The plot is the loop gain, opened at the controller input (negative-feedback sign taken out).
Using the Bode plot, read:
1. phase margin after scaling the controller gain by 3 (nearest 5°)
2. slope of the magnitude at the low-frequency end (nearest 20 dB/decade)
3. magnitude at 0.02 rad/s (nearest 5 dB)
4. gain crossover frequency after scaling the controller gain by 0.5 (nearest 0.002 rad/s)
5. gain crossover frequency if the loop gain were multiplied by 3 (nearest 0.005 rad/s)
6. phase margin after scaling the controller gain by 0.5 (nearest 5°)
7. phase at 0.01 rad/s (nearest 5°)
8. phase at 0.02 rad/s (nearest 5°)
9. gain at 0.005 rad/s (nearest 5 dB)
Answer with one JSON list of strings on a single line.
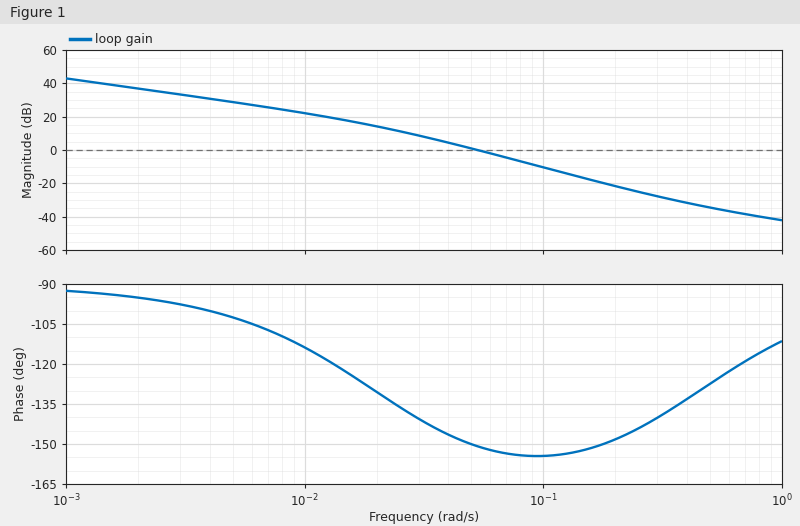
["25°", "-20 dB/decade", "15 dB", "0.036 rad/s", "0.095 rad/s", "35°", "-115°", "-130°", "30 dB"]
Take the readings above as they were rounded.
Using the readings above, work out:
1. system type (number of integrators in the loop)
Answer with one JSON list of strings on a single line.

["1"]
